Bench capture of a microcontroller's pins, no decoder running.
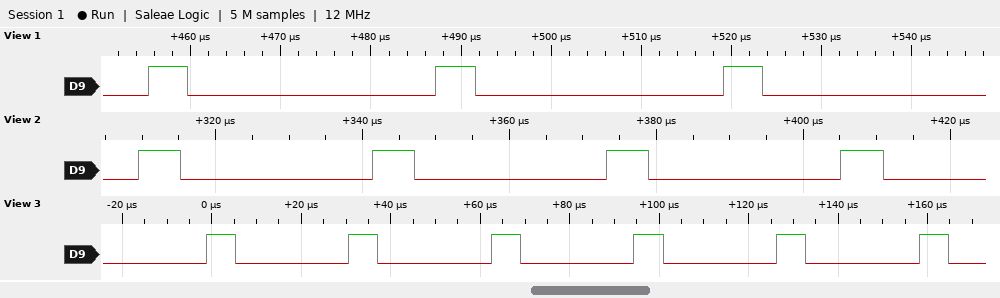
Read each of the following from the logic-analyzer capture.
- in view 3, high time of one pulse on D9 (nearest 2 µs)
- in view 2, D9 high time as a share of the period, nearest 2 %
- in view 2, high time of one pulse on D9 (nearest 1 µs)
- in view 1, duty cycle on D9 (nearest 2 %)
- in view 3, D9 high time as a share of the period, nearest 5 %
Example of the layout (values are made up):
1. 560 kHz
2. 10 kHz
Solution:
1. 6 µs
2. 18 %
3. 6 µs
4. 14 %
5. 20 %
